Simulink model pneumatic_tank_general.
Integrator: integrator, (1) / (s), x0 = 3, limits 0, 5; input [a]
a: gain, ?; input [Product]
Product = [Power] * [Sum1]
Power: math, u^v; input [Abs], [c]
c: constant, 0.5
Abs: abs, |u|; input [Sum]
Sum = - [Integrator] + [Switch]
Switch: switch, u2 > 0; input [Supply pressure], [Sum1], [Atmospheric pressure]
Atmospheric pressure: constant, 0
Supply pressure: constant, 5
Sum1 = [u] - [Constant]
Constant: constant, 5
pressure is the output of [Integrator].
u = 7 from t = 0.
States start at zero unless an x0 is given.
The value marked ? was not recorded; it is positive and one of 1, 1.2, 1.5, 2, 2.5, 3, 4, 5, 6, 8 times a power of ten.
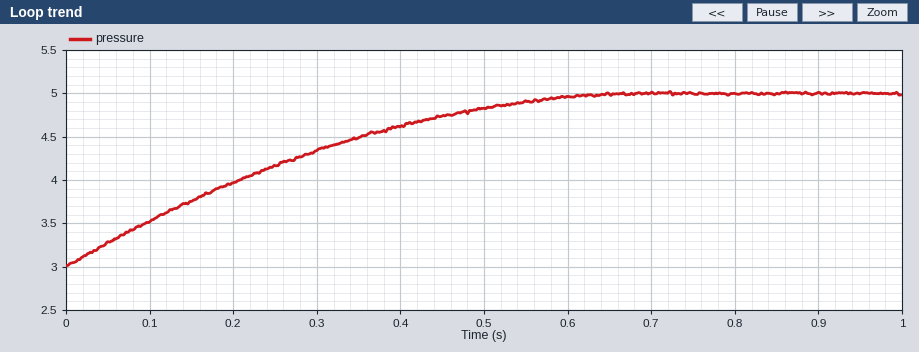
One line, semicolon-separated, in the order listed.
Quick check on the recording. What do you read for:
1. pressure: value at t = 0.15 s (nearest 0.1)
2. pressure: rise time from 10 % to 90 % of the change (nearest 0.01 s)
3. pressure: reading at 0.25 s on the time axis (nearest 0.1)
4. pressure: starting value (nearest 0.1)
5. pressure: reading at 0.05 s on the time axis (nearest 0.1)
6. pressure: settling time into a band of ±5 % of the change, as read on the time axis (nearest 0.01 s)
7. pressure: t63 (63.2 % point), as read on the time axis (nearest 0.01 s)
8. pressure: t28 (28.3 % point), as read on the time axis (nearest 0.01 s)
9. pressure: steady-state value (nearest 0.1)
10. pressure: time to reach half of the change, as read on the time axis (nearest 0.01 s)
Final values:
3.8; 0.45 s; 4.2; 3.0; 3.3; 0.55 s; 0.28 s; 0.11 s; 5.0; 0.21 s
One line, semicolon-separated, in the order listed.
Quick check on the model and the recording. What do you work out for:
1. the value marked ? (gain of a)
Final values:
2
